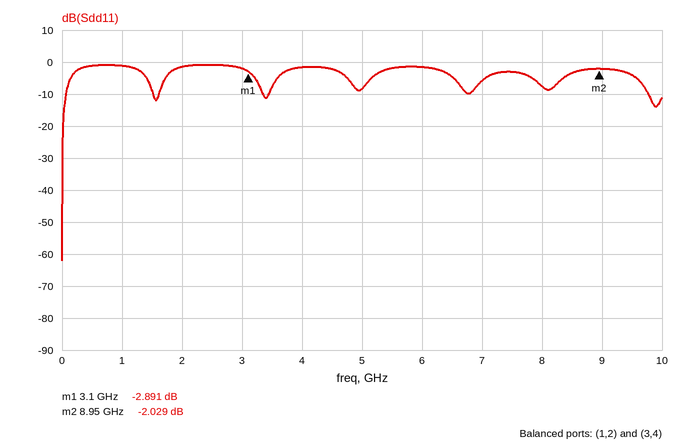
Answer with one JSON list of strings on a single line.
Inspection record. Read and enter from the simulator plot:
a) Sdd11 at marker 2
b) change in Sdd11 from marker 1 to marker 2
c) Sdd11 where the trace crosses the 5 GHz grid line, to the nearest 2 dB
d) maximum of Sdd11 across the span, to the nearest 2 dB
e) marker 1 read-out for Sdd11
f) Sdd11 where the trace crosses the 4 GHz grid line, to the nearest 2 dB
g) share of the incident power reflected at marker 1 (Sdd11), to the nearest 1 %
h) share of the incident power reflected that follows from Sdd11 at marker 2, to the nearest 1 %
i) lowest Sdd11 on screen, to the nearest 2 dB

["-2.029 dB", "0.862 dB", "-8 dB", "0 dB", "-2.891 dB", "-2 dB", "51 %", "63 %", "-62 dB"]
